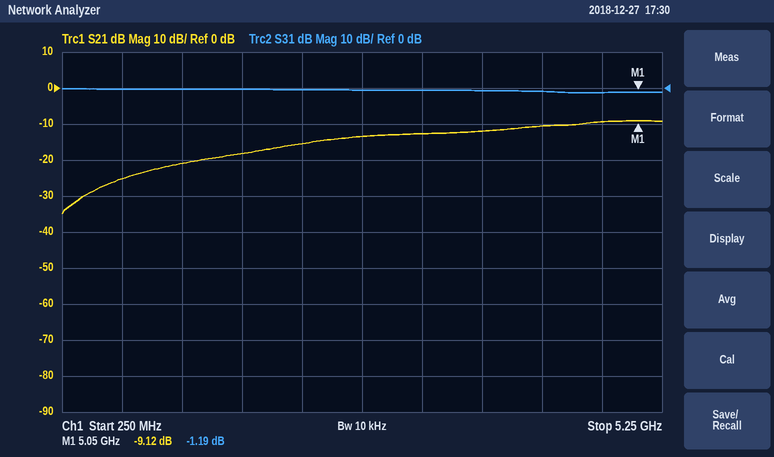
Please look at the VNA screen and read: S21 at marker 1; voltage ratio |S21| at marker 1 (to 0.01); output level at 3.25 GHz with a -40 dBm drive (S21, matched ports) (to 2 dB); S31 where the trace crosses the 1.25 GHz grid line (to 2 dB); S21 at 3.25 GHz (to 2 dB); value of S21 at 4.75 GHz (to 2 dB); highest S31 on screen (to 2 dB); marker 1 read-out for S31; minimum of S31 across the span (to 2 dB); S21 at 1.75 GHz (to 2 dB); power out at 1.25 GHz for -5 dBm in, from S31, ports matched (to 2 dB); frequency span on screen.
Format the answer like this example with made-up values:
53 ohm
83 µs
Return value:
-9.12 dB
0.35
-52 dBm
0 dB
-12 dB
-10 dB
0 dB
-1.19 dB
-2 dB
-18 dB
-6 dBm
5 GHz
